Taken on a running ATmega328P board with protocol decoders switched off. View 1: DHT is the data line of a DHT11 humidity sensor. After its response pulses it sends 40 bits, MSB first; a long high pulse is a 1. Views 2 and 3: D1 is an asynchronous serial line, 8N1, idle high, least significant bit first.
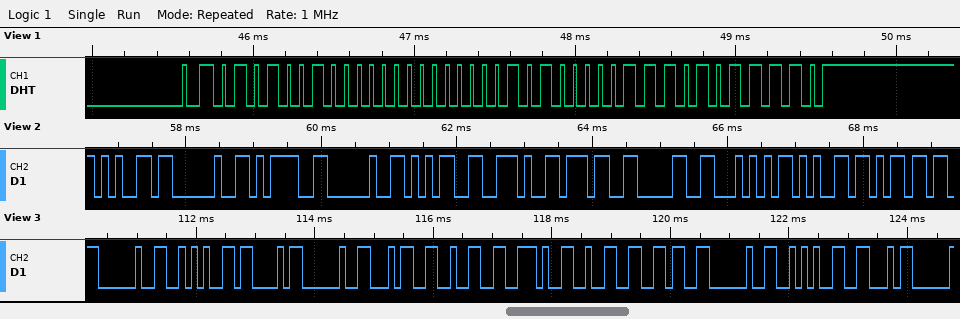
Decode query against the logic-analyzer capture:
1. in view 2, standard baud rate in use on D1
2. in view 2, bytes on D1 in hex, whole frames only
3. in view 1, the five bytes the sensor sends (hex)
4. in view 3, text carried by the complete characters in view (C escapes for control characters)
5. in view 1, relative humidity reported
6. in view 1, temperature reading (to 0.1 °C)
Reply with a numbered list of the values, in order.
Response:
1. 9600 baud
2. 65 20 3D 20 35 2E 37 30 54 65 6D
3. 52 00 05 07 5E
4. " *C 42.26 *F"
5. 82 %
6. 5.7 °C
